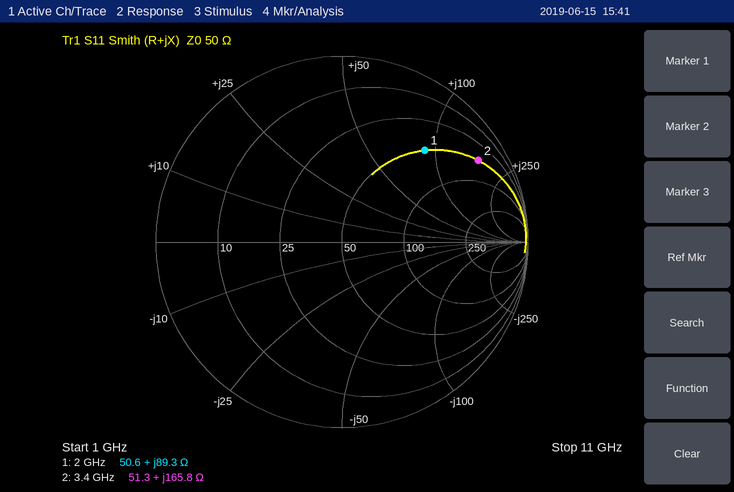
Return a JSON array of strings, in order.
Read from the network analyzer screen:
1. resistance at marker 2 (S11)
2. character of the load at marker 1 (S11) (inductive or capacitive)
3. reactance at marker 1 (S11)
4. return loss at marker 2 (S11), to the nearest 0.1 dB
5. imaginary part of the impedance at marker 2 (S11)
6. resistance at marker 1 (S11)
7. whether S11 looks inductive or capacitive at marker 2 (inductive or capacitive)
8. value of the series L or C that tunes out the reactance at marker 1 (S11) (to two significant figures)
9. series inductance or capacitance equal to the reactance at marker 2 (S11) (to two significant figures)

["51.3 Ω", "inductive", "+89.3 Ω", "1.4 dB", "+165.8 Ω", "50.6 Ω", "inductive", "890 fF", "7.8 nH"]
